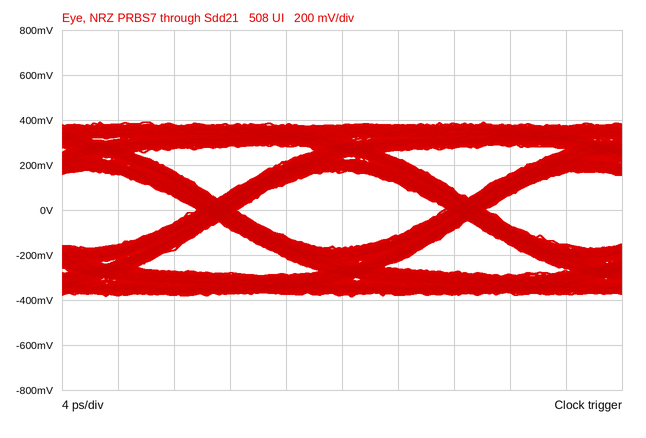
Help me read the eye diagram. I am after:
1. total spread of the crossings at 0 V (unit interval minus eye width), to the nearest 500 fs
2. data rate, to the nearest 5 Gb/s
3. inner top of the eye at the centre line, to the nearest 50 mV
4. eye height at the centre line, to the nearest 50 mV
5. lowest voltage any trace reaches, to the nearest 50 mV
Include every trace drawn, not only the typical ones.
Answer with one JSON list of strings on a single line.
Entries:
["3.0 ps", "55 Gb/s", "150 mV", "350 mV", "-400 mV"]
